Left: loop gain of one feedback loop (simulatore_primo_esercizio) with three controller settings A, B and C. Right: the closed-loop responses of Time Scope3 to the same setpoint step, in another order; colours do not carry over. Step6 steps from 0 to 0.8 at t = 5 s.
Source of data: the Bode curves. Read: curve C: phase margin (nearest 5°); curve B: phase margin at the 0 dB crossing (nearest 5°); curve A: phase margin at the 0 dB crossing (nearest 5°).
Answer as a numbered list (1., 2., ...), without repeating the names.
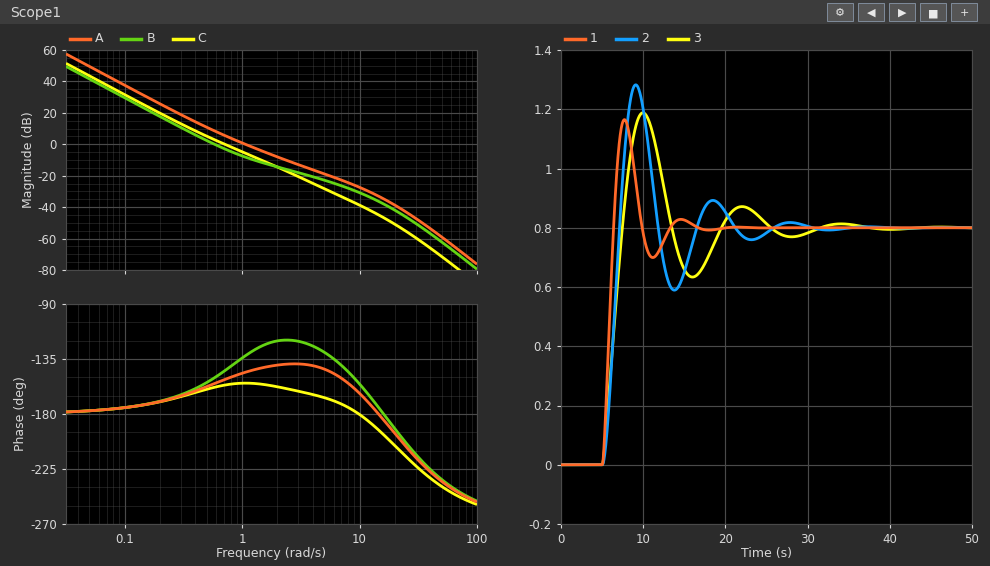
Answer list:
1. 25°
2. 30°
3. 35°
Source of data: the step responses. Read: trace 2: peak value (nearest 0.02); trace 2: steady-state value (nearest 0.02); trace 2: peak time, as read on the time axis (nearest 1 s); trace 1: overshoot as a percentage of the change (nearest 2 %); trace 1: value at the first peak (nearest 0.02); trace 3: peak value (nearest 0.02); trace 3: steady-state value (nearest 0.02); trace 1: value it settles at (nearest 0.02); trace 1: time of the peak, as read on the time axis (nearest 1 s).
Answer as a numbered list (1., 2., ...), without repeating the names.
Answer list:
1. 1.28
2. 0.80
3. 9 s
4. 46 %
5. 1.16
6. 1.18
7. 0.80
8. 0.80
9. 8 s
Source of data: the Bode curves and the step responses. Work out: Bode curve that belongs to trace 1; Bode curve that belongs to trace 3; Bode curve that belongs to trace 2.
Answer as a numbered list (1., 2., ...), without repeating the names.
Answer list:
1. A
2. B
3. C
